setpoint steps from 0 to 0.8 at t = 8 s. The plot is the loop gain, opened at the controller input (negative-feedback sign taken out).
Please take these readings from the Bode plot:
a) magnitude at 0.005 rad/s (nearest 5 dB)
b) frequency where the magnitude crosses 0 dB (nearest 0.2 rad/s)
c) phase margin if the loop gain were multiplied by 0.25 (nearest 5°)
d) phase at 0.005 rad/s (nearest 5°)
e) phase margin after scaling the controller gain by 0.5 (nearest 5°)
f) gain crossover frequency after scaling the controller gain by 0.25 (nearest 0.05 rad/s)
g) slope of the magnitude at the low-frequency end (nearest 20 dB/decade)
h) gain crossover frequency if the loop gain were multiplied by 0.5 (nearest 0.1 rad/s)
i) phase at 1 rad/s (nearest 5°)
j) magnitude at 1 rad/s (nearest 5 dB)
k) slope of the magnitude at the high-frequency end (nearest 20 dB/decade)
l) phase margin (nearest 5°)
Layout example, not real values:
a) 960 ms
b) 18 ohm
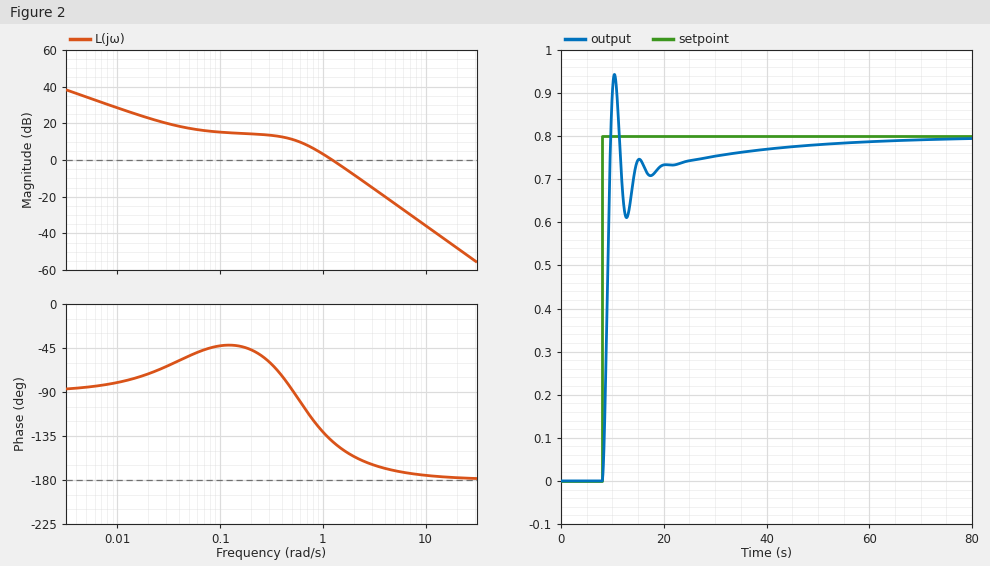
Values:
a) 35 dB
b) 1.2 rad/s
c) 100°
d) -85°
e) 60°
f) 0.45 rad/s
g) -20 dB/decade
h) 0.8 rad/s
i) -130°
j) 5 dB
k) -40 dB/decade
l) 40°
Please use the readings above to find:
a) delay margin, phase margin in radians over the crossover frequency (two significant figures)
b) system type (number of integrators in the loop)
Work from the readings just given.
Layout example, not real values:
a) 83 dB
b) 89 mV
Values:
a) 0.58 s
b) 1
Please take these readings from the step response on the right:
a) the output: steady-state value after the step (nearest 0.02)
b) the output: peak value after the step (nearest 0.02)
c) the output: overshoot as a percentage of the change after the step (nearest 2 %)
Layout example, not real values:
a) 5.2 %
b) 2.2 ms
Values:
a) 0.80
b) 0.94
c) 18 %
